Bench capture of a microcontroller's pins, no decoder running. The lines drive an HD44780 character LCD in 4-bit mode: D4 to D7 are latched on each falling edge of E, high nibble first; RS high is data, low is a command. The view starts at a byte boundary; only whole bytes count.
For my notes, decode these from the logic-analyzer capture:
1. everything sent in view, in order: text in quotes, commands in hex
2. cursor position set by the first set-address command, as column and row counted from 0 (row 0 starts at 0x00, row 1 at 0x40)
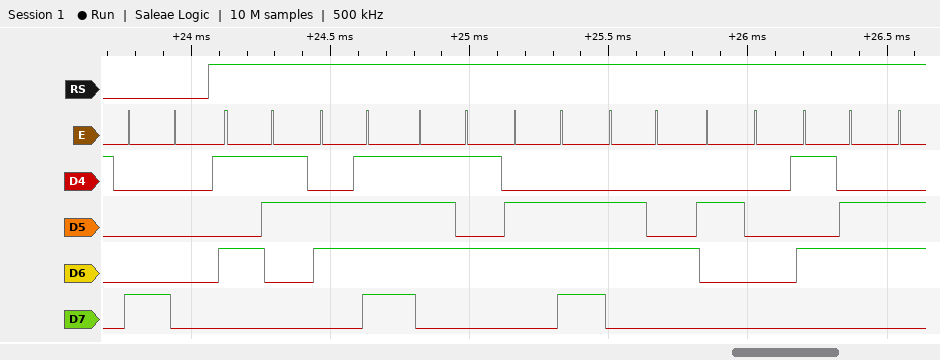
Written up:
0x80 "Sound V"
column 0, row 0
